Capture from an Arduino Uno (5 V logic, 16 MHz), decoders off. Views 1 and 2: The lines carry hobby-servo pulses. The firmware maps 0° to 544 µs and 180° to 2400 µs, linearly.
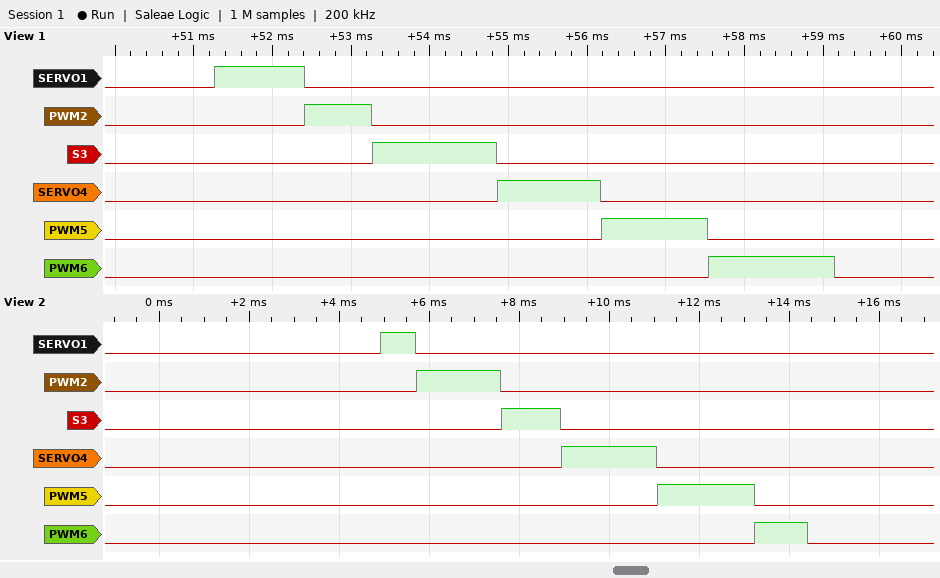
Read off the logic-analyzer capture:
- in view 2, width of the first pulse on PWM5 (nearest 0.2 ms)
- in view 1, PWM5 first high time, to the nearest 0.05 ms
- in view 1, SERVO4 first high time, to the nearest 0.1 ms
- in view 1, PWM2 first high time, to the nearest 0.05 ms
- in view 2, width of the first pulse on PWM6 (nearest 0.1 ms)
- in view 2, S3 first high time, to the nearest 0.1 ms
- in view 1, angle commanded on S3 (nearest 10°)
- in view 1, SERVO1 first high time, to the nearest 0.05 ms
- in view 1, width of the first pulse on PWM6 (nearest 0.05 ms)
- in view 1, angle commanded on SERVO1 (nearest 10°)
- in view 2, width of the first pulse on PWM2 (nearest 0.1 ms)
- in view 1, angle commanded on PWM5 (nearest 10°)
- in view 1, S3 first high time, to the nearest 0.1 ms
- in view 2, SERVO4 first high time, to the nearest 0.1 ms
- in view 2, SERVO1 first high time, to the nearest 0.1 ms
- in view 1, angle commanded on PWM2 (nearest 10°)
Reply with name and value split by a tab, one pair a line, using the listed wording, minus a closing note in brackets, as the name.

in view 2, width of the first pulse on PWM5	2.2 ms
in view 1, PWM5 first high time, to the nearest 0.05 ms	1.35 ms
in view 1, SERVO4 first high time, to the nearest 0.1 ms	1.3 ms
in view 1, PWM2 first high time, to the nearest 0.05 ms	0.85 ms
in view 2, width of the first pulse on PWM6	1.2 ms
in view 2, S3 first high time, to the nearest 0.1 ms	1.3 ms
in view 1, angle commanded on S3	100°
in view 1, SERVO1 first high time, to the nearest 0.05 ms	1.15 ms
in view 1, width of the first pulse on PWM6	1.60 ms
in view 1, angle commanded on SERVO1	60°
in view 2, width of the first pulse on PWM2	1.9 ms
in view 1, angle commanded on PWM5	80°
in view 1, S3 first high time, to the nearest 0.1 ms	1.6 ms
in view 2, SERVO4 first high time, to the nearest 0.1 ms	2.1 ms
in view 2, SERVO1 first high time, to the nearest 0.1 ms	0.8 ms
in view 1, angle commanded on PWM2	30°
